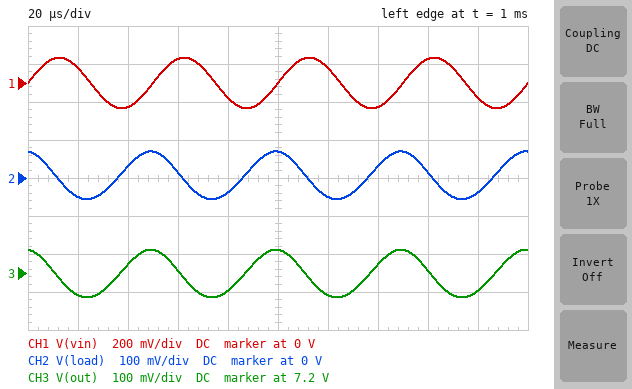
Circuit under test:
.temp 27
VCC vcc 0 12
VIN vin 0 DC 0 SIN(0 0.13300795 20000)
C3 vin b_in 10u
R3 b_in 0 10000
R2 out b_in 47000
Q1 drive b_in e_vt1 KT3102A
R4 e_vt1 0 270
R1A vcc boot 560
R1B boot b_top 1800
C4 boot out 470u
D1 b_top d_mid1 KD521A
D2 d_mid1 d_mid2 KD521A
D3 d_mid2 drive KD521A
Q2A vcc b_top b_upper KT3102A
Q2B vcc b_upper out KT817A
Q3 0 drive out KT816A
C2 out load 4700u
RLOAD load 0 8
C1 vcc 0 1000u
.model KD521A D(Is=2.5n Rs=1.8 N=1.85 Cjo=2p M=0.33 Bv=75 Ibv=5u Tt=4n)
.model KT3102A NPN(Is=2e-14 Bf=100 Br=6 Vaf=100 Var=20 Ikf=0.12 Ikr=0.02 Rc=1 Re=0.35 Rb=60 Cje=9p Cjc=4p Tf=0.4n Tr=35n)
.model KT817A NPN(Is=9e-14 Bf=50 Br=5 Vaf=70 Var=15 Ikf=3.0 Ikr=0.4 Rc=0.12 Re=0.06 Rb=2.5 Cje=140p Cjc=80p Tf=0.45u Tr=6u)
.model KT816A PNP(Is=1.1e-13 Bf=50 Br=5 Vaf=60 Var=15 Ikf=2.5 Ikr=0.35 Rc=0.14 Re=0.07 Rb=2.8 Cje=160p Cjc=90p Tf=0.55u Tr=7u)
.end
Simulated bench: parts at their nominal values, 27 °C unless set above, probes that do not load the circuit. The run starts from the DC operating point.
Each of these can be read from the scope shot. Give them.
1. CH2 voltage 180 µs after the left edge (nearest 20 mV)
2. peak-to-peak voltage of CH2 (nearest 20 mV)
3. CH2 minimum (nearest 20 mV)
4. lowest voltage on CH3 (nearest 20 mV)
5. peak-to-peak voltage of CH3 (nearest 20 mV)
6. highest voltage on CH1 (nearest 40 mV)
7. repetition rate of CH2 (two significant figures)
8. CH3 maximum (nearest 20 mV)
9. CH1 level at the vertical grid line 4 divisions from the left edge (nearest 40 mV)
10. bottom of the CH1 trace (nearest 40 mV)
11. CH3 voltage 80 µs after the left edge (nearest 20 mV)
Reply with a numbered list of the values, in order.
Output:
1. -40 mV
2. 120 mV
3. -60 mV
4. 7.14 V
5. 120 mV
6. 120 mV
7. 20 kHz
8. 7.26 V
9. -80 mV
10. -120 mV
11. 7.16 V
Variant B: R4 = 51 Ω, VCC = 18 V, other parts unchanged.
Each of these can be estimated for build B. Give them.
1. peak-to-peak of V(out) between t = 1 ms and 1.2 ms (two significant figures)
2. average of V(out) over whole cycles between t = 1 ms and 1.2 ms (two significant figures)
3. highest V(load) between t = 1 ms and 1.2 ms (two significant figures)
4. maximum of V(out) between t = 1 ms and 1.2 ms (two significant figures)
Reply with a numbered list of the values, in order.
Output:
1. 660 mV
2. 7.8 V
3. 350 mV
4. 8.1 V
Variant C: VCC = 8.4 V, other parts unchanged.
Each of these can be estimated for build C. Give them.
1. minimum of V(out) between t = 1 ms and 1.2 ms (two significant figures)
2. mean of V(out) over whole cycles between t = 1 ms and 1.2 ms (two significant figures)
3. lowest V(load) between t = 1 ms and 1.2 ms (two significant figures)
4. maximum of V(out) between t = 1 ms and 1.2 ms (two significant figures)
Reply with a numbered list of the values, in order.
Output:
1. 5.4 V
2. 5.6 V
3. 89 mV
4. 6.0 V
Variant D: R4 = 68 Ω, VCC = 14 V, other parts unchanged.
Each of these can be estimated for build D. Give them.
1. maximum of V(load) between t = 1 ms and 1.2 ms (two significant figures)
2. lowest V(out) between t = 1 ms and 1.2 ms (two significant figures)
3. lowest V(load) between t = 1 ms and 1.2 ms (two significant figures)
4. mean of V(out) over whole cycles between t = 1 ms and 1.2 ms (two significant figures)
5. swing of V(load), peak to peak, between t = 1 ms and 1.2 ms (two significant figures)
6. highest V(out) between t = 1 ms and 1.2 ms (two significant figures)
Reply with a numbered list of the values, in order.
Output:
1. 270 mV
2. 6.4 V
3. -210 mV
4. 6.6 V
5. 480 mV
6. 6.9 V
